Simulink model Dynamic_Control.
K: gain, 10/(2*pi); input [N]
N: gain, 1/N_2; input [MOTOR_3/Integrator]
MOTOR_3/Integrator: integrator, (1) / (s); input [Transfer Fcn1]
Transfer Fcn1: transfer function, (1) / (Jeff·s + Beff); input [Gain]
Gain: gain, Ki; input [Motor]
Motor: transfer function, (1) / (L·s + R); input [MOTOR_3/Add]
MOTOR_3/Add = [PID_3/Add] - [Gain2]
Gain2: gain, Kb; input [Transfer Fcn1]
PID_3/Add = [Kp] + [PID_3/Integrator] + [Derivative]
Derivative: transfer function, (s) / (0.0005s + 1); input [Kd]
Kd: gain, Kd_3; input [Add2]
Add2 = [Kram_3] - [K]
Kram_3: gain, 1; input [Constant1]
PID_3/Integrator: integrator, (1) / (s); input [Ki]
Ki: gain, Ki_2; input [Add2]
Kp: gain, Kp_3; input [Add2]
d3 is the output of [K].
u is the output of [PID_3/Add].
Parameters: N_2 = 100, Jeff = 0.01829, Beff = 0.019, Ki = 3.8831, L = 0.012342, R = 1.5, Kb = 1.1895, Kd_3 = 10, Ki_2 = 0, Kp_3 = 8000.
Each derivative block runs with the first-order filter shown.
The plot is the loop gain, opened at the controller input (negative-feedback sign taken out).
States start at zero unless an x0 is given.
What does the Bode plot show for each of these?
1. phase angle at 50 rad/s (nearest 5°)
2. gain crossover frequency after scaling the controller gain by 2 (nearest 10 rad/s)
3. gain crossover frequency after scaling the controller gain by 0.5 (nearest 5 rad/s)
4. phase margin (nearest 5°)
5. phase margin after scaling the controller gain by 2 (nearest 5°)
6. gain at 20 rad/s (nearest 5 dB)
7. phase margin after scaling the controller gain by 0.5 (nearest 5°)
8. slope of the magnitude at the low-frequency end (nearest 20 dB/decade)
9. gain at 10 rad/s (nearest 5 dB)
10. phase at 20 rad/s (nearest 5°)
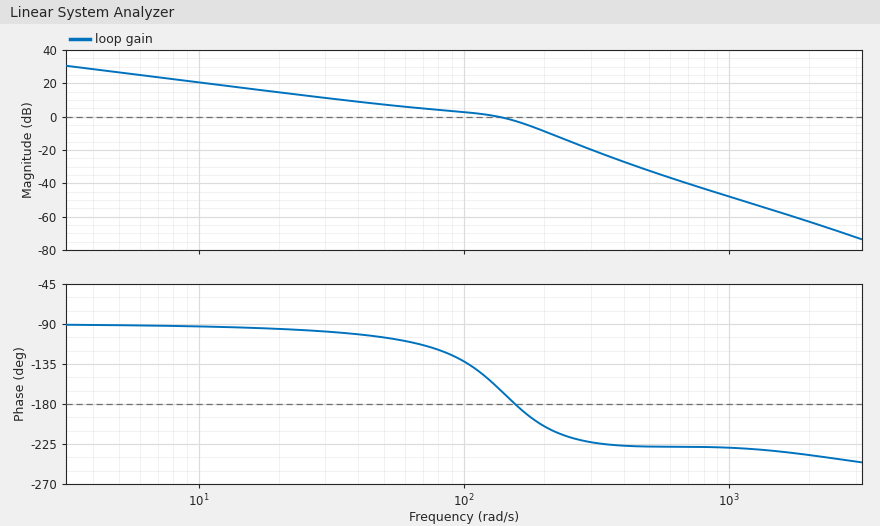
-105°
180 rad/s
60 rad/s
20°
-15°
15 dB
70°
-20 dB/decade
20 dB
-95°
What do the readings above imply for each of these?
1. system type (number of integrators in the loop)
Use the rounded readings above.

1
